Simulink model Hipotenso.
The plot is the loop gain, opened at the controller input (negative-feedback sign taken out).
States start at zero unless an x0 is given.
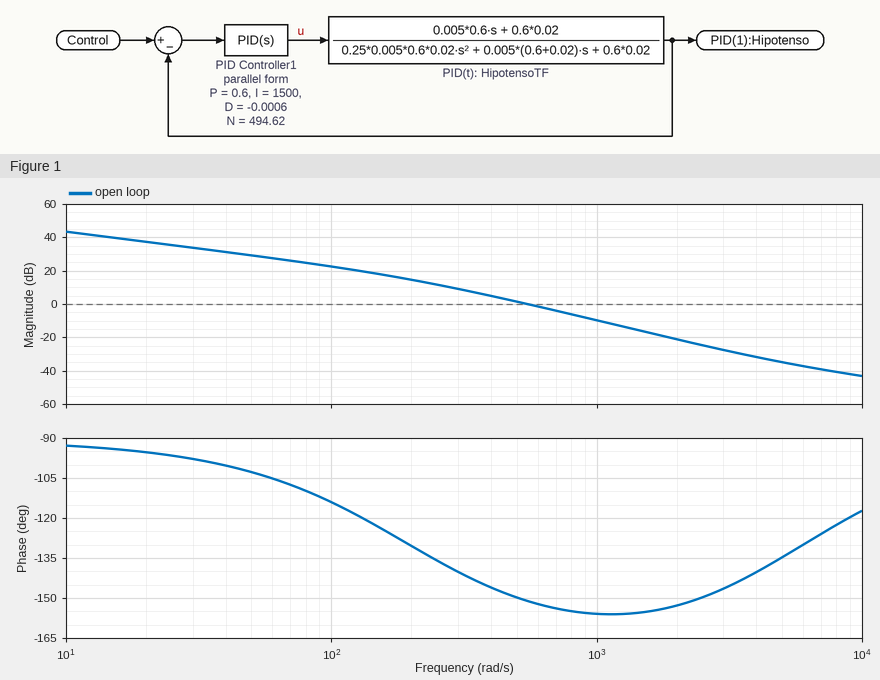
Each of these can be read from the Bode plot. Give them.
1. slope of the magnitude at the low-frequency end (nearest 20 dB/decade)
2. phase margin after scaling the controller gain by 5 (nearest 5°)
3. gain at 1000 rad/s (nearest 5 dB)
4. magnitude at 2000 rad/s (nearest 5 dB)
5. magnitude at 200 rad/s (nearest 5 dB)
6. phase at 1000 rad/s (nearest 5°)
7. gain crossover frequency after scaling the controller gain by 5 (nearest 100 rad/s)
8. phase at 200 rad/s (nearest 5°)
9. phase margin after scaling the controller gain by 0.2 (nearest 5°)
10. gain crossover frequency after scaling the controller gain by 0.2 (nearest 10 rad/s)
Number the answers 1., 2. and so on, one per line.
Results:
1. -20 dB/decade
2. 25°
3. -10 dB
4. -20 dB
5. 15 dB
6. -155°
7. 1300 rad/s
8. -130°
9. 50°
10. 210 rad/s
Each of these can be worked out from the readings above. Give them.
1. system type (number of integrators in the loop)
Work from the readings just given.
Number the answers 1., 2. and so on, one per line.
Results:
1. 1
